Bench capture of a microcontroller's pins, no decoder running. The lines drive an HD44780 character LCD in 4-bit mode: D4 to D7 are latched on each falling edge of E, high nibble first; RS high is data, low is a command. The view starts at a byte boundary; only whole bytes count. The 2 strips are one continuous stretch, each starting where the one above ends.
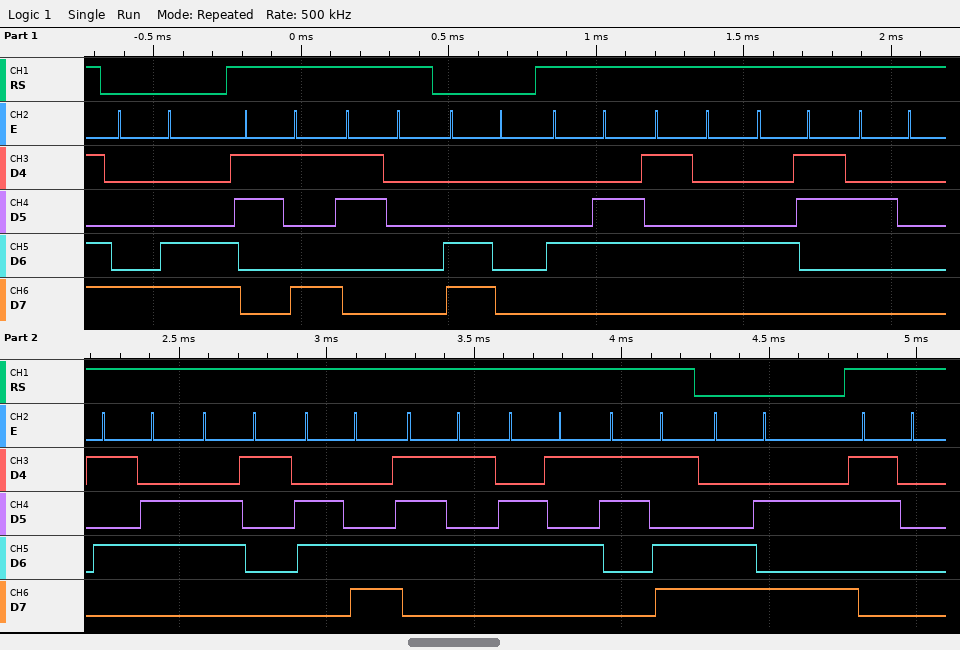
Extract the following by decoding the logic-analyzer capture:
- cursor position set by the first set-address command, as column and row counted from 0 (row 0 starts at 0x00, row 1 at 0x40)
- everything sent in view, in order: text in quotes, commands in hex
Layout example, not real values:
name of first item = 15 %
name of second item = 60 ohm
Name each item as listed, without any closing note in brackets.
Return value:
cursor position set by the first set-address command, as column and row counted from 0 = column 12, row 0
everything sent in view, in order: text in quotes, commands in hex = 0x8C "90" 0xC0 "FTC Value=" 0xCA "0"
